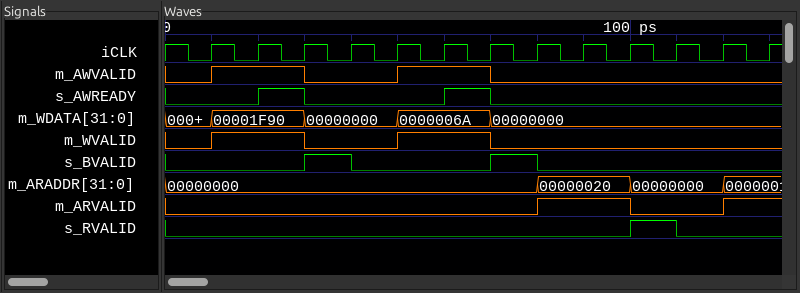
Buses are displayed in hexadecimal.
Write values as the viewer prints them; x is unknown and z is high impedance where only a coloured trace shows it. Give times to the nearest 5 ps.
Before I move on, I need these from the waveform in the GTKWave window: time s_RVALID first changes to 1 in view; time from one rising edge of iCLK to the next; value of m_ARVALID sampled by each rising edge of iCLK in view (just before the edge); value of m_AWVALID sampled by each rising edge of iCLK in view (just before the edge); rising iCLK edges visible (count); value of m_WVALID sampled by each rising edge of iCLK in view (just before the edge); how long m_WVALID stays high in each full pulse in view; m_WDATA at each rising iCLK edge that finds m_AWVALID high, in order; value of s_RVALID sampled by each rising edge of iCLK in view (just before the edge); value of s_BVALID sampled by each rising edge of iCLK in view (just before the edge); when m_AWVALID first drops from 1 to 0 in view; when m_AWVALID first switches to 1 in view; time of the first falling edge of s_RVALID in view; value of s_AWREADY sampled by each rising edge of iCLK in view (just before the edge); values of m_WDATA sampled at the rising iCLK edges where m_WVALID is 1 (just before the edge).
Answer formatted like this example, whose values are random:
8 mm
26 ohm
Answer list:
100 ps
10 ps
0 0 0 0 0 0 0 0 1 1 0 0 1
0 1 1 0 0 1 1 0 0 0 0 0 0
13
0 1 1 0 0 1 1 0 0 0 0 0 0
20 ps, 20 ps
00001F90, 00001F90, 0000006A, 0000006A
0 0 0 0 0 0 0 0 0 0 1 0 0
0 0 0 1 0 0 0 1 0 0 0 0 0
30 ps
10 ps
110 ps
0 0 1 0 0 0 1 0 0 0 0 0 0
00001F90, 00001F90, 0000006A, 0000006A
